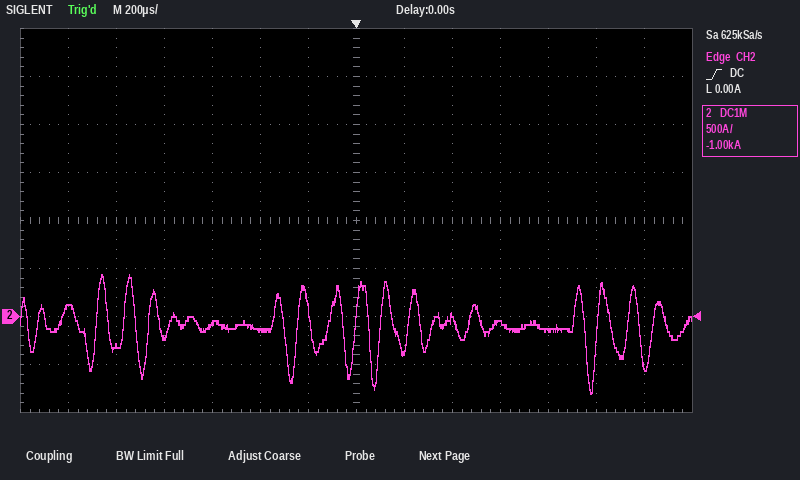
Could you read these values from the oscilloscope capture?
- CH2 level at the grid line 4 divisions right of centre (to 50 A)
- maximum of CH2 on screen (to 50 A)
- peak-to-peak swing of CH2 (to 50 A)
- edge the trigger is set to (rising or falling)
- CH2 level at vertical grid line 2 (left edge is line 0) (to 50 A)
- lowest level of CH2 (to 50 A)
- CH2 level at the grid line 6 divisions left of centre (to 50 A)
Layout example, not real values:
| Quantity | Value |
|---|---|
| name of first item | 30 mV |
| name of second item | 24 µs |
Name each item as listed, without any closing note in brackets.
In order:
| Quantity | Value |
|---|---|
| CH2 level at the grid line 4 divisions right of centre | -150 A |
| maximum of CH2 on screen | 450 A |
| peak-to-peak swing of CH2 | 1.25 kA |
| edge the trigger is set to | rising |
| CH2 level at vertical grid line 2 (left edge is line 0) | -300 A |
| lowest level of CH2 | -800 A |
| CH2 level at the grid line 6 divisions left of centre | 100 A |
